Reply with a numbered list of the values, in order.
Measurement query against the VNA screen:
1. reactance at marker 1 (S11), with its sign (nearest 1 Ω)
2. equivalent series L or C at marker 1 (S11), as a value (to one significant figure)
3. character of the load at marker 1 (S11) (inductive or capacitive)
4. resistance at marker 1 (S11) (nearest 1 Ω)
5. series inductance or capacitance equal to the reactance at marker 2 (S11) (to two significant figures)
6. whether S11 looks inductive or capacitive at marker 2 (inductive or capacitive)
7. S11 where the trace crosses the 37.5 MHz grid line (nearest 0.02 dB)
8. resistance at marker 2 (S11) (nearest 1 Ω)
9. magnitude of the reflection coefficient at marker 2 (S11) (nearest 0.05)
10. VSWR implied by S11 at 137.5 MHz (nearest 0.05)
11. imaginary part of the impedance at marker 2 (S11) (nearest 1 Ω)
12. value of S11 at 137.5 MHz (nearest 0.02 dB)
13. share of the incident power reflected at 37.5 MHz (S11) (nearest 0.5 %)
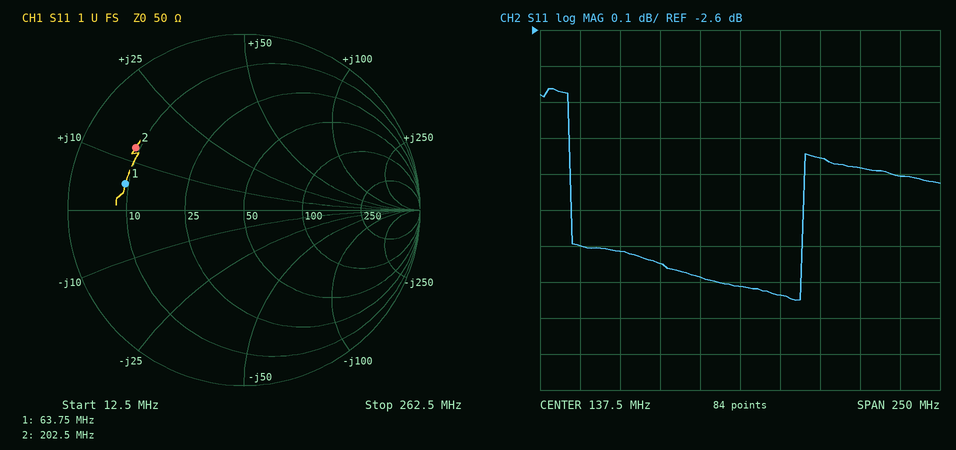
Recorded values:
1. +5 Ω
2. 10 nH
3. inductive
4. 9 Ω
5. 10 nH
6. inductive
7. -3.20 dB
8. 9 Ω
9. 0.70
10. 5.30
11. +13 Ω
12. -3.32 dB
13. 48.0 %
